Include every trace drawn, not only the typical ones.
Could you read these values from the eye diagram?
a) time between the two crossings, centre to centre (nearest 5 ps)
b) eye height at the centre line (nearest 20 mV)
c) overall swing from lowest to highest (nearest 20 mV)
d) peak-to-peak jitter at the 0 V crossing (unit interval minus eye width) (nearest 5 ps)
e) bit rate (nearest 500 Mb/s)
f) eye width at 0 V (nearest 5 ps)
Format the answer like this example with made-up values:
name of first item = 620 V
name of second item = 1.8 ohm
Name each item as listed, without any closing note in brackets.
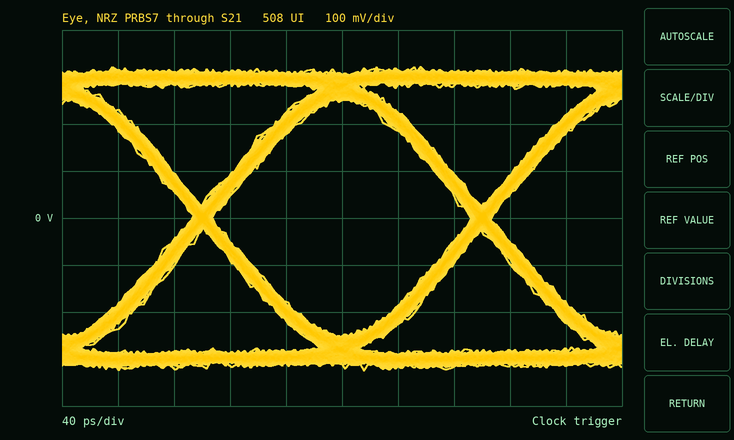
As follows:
time between the two crossings, centre to centre = 200 ps
eye height at the centre line = 500 mV
overall swing from lowest to highest = 640 mV
peak-to-peak jitter at the 0 V crossing (unit interval minus eye width) = 15 ps
bit rate = 5.0 Gb/s
eye width at 0 V = 185 ps
